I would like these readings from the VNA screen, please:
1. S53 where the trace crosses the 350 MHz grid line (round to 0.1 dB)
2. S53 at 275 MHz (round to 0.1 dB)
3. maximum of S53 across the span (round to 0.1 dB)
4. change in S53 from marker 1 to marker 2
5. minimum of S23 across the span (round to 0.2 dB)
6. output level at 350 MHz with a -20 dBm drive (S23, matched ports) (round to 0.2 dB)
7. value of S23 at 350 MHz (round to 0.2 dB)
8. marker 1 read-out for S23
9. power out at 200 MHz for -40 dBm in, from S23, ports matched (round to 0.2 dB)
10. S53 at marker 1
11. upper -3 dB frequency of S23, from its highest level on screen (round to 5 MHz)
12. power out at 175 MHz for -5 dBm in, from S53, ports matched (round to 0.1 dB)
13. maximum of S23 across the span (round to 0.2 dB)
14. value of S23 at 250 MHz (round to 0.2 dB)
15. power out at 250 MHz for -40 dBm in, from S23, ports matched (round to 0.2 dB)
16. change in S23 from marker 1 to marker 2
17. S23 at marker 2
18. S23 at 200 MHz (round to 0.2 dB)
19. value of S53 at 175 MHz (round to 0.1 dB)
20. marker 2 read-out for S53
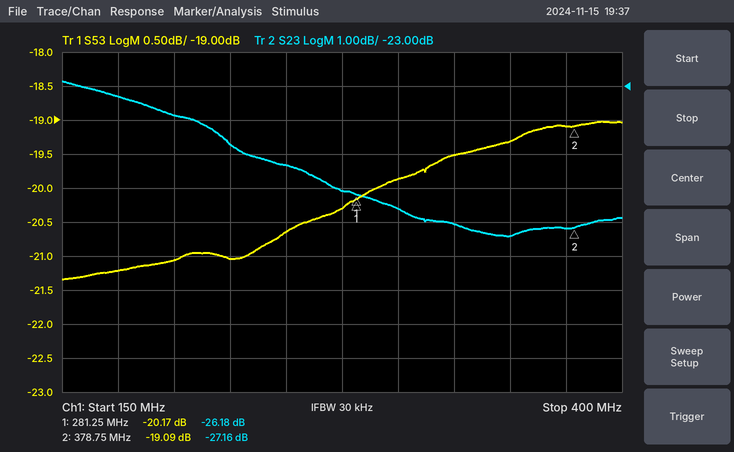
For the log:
-19.3 dB
-20.3 dB
-19.0 dB
1.08 dB
-27.4 dB
-47.4 dBm
-27.4 dB
-26.18 dB
-63.8 dBm
-20.17 dB
270 MHz
-26.2 dBm
-22.8 dB
-25.4 dB
-65.4 dBm
-0.98 dB
-27.16 dB
-23.8 dB
-21.2 dB
-19.09 dB
